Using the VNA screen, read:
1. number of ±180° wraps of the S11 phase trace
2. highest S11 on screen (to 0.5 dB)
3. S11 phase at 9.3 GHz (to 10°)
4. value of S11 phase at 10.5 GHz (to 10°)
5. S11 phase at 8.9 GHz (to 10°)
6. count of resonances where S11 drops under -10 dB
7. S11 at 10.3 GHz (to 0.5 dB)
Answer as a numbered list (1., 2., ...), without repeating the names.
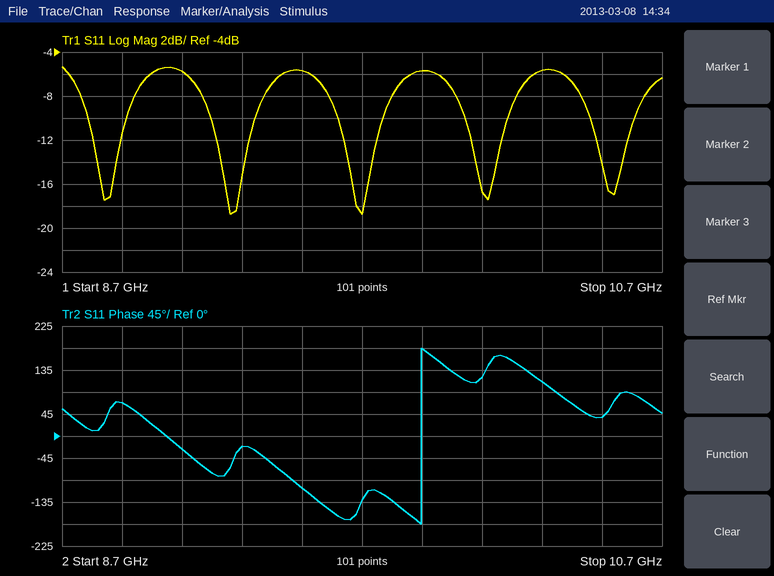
1. 1
2. -5.5 dB
3. -20°
4. 40°
5. 70°
6. 5
7. -5.5 dB
